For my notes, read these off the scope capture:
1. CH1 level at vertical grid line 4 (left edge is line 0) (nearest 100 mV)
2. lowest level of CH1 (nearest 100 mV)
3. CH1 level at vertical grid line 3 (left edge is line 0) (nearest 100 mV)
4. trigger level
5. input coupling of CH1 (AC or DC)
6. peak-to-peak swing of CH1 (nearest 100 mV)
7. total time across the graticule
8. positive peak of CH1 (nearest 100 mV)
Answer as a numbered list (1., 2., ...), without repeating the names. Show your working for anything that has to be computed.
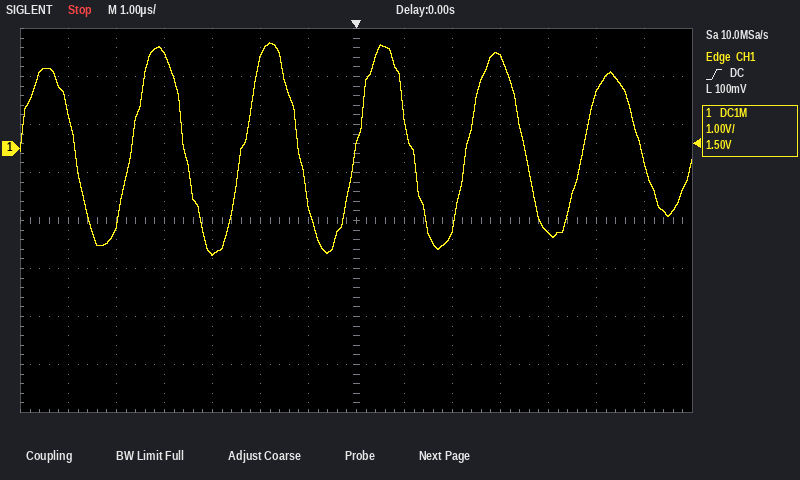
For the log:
1. -2.2 V
2. -2.2 V
3. 2.0 V
4. 100 mV
5. DC
6. 2.2 V − (-2.2 V) = 4.4 V
7. 14 µs
8. 2.2 V
